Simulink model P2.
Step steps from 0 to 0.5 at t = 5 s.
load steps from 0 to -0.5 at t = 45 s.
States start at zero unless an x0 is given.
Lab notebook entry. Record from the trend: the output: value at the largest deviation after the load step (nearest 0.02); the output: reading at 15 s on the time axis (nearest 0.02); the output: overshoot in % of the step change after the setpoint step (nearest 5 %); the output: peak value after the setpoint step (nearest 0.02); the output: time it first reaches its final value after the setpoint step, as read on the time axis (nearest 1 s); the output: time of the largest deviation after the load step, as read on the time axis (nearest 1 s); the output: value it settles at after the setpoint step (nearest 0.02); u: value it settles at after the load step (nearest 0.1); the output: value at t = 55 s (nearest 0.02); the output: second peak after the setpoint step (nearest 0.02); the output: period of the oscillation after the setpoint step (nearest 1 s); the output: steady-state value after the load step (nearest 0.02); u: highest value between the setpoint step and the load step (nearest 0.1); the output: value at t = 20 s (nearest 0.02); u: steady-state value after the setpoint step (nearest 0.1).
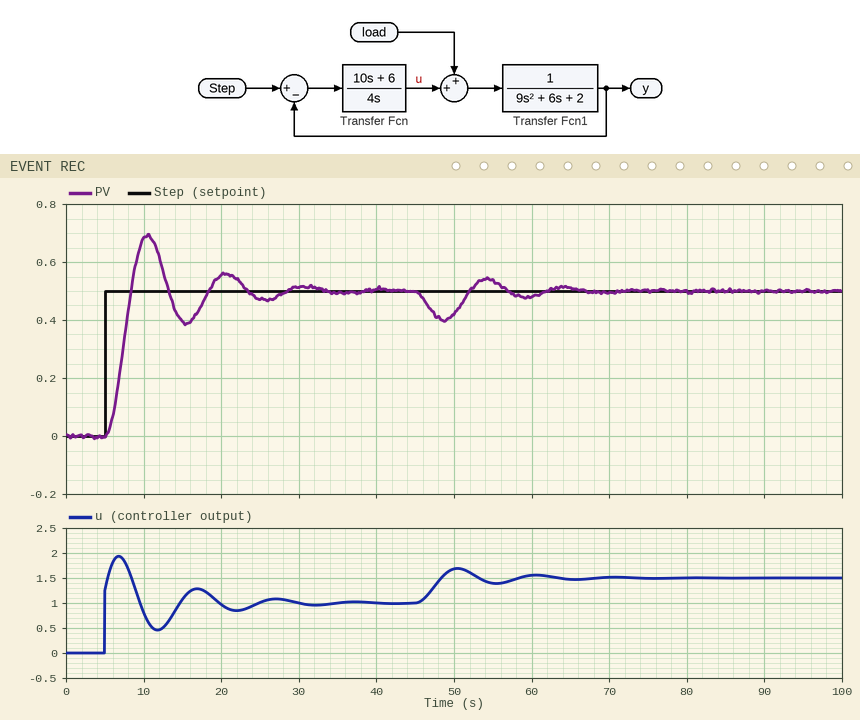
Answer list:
0.40
0.40
40 %
0.70
8 s
49 s
0.50
1.5
0.54
0.56
10 s
0.50
1.9
0.56
1.0
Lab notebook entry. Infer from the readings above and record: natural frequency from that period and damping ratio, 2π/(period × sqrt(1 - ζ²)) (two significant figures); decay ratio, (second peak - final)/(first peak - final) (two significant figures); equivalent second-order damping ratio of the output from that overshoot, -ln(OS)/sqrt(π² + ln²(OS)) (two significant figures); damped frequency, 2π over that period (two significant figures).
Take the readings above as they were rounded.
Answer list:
0.65 rad/s
0.30
0.28
0.63 rad/s
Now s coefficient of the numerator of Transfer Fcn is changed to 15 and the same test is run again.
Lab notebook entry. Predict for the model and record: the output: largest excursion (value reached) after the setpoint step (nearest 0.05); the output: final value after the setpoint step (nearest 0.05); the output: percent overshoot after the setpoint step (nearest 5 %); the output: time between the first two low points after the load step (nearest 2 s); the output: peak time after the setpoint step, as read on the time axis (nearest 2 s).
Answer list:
0.65
0.50
30 %
10 s
10 s
